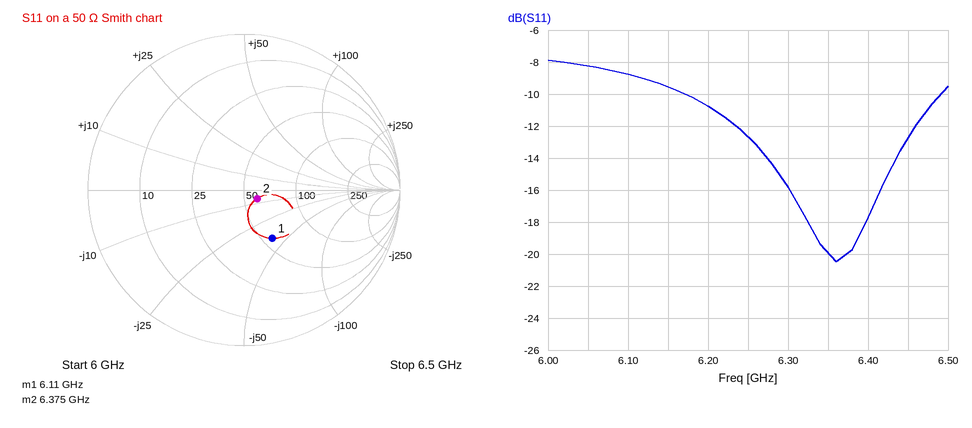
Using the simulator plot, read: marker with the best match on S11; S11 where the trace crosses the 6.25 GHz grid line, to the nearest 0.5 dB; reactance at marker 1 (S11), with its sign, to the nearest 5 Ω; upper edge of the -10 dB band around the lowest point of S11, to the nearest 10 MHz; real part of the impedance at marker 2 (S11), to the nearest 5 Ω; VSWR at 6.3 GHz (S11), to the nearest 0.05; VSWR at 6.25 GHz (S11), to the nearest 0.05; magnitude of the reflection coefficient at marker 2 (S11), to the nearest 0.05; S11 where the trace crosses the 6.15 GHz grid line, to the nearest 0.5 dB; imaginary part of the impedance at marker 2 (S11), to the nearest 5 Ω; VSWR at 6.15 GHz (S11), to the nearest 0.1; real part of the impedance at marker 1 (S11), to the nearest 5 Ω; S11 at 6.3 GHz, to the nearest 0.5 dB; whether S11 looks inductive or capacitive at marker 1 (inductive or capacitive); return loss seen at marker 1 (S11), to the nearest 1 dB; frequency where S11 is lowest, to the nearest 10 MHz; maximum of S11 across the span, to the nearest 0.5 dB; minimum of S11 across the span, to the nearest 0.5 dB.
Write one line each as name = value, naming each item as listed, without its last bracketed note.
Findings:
marker with the best match on S11 = marker 2
S11 where the trace crosses the 6.25 GHz grid line, to the nearest 0.5 dB = -12.5 dB
reactance at marker 1 (S11), with its sign, to the nearest 5 Ω = -40 Ω
upper edge of the -10 dB band around the lowest point of S11, to the nearest 10 MHz = 6.49 GHz
real part of the impedance at marker 2 (S11), to the nearest 5 Ω = 60 Ω
VSWR at 6.3 GHz (S11), to the nearest 0.05 = 1.40
VSWR at 6.25 GHz (S11), to the nearest 0.05 = 1.60
magnitude of the reflection coefficient at marker 2 (S11), to the nearest 0.05 = 0.10
S11 where the trace crosses the 6.15 GHz grid line, to the nearest 0.5 dB = -9.5 dB
imaginary part of the impedance at marker 2 (S11), to the nearest 5 Ω = -5 Ω
VSWR at 6.15 GHz (S11), to the nearest 0.1 = 2.0
real part of the impedance at marker 1 (S11), to the nearest 5 Ω = 55 Ω
S11 at 6.3 GHz, to the nearest 0.5 dB = -16.0 dB
whether S11 looks inductive or capacitive at marker 1 = capacitive
return loss seen at marker 1 (S11), to the nearest 1 dB = 9 dB
frequency where S11 is lowest, to the nearest 10 MHz = 6.36 GHz
maximum of S11 across the span, to the nearest 0.5 dB = -8.0 dB
minimum of S11 across the span, to the nearest 0.5 dB = -20.5 dB
